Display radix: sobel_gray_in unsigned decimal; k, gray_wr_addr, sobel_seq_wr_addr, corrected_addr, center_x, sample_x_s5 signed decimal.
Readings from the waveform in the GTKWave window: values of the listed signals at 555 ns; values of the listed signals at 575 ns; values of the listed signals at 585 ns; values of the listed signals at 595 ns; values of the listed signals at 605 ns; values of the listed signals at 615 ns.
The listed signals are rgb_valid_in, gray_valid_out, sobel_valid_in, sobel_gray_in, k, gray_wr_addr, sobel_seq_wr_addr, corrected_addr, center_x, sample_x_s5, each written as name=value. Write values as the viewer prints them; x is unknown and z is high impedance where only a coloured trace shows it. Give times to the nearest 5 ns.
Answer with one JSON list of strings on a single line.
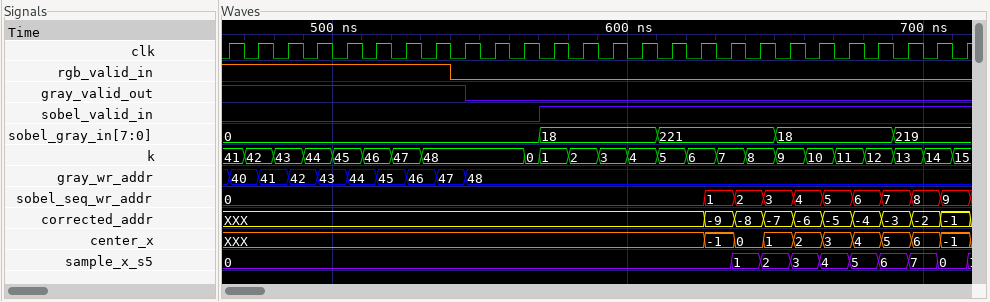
["rgb_valid_in=0, gray_valid_out=0, sobel_valid_in=0, sobel_gray_in=0, k=48, gray_wr_addr=48, sobel_seq_wr_addr=0, corrected_addr=XXX, center_x=XXX, sample_x_s5=0", "rgb_valid_in=0, gray_valid_out=0, sobel_valid_in=1, sobel_gray_in=18, k=1, gray_wr_addr=48, sobel_seq_wr_addr=0, corrected_addr=XXX, center_x=XXX, sample_x_s5=0", "rgb_valid_in=0, gray_valid_out=0, sobel_valid_in=1, sobel_gray_in=18, k=2, gray_wr_addr=48, sobel_seq_wr_addr=0, corrected_addr=XXX, center_x=XXX, sample_x_s5=0", "rgb_valid_in=0, gray_valid_out=0, sobel_valid_in=1, sobel_gray_in=18, k=3, gray_wr_addr=48, sobel_seq_wr_addr=0, corrected_addr=XXX, center_x=XXX, sample_x_s5=0", "rgb_valid_in=0, gray_valid_out=0, sobel_valid_in=1, sobel_gray_in=18, k=4, gray_wr_addr=48, sobel_seq_wr_addr=0, corrected_addr=XXX, center_x=XXX, sample_x_s5=0", "rgb_valid_in=0, gray_valid_out=0, sobel_valid_in=1, sobel_gray_in=221, k=5, gray_wr_addr=48, sobel_seq_wr_addr=0, corrected_addr=XXX, center_x=XXX, sample_x_s5=0"]
